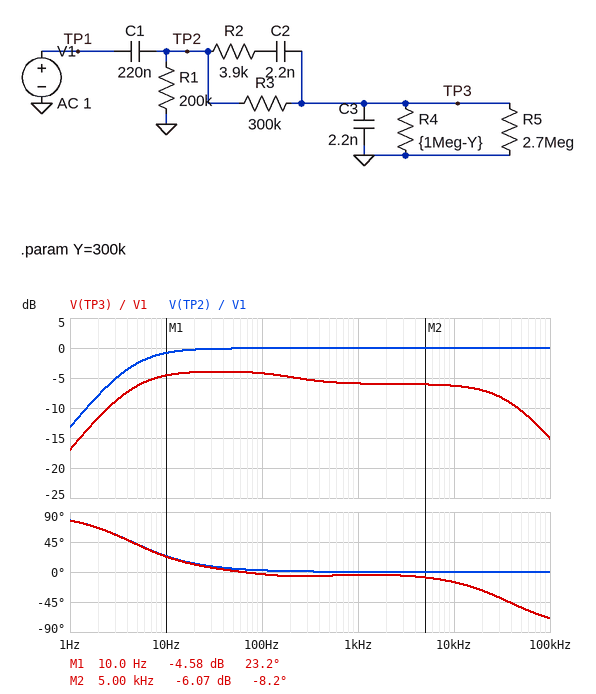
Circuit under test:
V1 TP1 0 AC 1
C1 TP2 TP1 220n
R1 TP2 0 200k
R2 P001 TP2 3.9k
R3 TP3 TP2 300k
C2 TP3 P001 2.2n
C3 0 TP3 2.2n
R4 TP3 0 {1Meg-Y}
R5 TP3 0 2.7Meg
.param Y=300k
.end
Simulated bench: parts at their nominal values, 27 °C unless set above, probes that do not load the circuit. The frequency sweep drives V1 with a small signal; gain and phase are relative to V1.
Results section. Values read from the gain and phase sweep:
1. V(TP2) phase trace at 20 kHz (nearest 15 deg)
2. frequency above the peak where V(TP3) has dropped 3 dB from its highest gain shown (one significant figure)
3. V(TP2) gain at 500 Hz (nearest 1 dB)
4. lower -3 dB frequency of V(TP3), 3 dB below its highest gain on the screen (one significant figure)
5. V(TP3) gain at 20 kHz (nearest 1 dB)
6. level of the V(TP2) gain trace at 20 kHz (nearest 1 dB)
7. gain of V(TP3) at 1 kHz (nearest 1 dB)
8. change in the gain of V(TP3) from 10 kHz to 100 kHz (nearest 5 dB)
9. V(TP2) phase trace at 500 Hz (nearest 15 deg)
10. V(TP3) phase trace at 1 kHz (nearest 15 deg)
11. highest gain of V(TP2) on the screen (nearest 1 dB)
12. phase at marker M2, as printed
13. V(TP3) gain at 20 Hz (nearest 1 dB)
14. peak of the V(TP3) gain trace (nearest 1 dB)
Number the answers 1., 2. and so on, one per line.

1. 0 deg
2. 20 kHz
3. 0 dB
4. 4 Hz
5. -7 dB
6. 0 dB
7. -6 dB
8. -10 dB
9. 0 deg
10. 0 deg
11. 0 dB
12. -8.2 deg
13. -4 dB
14. -4 dB
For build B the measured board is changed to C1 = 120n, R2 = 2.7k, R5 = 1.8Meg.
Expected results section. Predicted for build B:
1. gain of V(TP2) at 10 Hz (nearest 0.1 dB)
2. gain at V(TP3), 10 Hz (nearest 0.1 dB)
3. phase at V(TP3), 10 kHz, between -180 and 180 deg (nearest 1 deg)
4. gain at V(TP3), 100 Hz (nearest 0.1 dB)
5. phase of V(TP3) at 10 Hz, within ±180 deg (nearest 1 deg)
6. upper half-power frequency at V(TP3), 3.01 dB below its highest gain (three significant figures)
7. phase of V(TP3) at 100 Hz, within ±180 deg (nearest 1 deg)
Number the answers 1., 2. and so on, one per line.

1. -2.3 dB
2. -6.4 dB
3. -11 deg
4. -4.5 dB
5. 39 deg
6. 32.2 kHz
7. 0 deg
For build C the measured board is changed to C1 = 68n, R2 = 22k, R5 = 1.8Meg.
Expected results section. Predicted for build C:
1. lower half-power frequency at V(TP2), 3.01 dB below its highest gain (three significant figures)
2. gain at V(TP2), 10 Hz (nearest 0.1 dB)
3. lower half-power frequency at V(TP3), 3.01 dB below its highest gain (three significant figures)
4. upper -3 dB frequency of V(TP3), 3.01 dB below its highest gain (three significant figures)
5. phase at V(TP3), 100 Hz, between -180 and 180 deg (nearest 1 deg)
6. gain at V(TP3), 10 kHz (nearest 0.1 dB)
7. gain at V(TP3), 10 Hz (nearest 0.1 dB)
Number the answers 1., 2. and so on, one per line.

1. 14.9 Hz
2. -5.0 dB
3. 13.3 Hz
4. 4.87 kHz
5. 3 deg
6. -10.7 dB
7. -9.1 dB
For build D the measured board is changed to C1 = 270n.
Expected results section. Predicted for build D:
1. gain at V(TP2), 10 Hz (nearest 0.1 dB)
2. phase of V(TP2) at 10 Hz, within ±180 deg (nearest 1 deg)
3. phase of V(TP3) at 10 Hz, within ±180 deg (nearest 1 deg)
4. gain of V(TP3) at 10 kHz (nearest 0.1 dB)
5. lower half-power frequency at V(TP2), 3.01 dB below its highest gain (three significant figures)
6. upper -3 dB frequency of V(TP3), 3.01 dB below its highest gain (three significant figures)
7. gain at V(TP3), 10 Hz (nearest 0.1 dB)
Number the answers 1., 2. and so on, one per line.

1. -0.6 dB
2. 20 deg
3. 19 deg
4. -6.3 dB
5. 3.65 Hz
6. 18.1 kHz
7. -4.3 dB
